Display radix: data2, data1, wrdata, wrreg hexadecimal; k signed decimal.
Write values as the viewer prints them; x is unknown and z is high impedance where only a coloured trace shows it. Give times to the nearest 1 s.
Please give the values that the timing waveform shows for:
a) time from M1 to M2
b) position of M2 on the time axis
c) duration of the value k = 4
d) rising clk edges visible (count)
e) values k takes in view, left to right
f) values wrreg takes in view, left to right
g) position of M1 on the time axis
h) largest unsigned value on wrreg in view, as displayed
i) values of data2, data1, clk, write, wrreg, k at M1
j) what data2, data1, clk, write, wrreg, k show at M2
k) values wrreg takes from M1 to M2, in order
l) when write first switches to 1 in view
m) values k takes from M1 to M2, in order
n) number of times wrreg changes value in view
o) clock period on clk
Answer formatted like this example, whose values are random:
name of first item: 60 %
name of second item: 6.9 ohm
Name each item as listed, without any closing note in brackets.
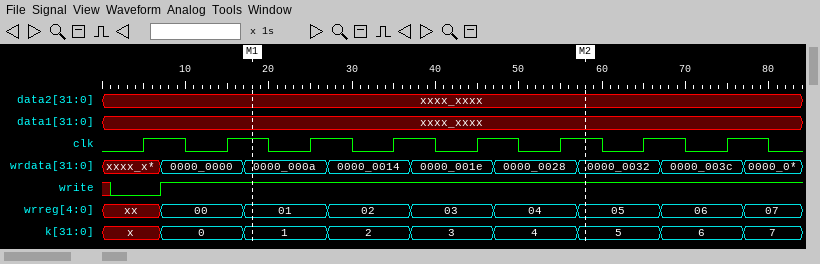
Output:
time from M1 to M2: 40 s
position of M2 on the time axis: 58 s
duration of the value k = 4: 10 s
rising clk edges visible: 8
values k takes in view, left to right: x, 0, 1, 2, 3, 4, 5, 6, 7
values wrreg takes in view, left to right: xx, 00, 01, 02, 03, 04, 05, 06, 07
position of M1 on the time axis: 18 s
largest unsigned value on wrreg in view, as displayed: 07
values of data2, data1, clk, write, wrreg, k at M1: data2=xxxx_xxxx, data1=xxxx_xxxx, clk=1, write=1, wrreg=01, k=1
what data2, data1, clk, write, wrreg, k show at M2: data2=xxxx_xxxx, data1=xxxx_xxxx, clk=1, write=1, wrreg=05, k=5
values wrreg takes from M1 to M2, in order: 01, 02, 03, 04, 05
when write first switches to 1 in view: 7 s
values k takes from M1 to M2, in order: 1, 2, 3, 4, 5
number of times wrreg changes value in view: 8
clock period on clk: 10 s
